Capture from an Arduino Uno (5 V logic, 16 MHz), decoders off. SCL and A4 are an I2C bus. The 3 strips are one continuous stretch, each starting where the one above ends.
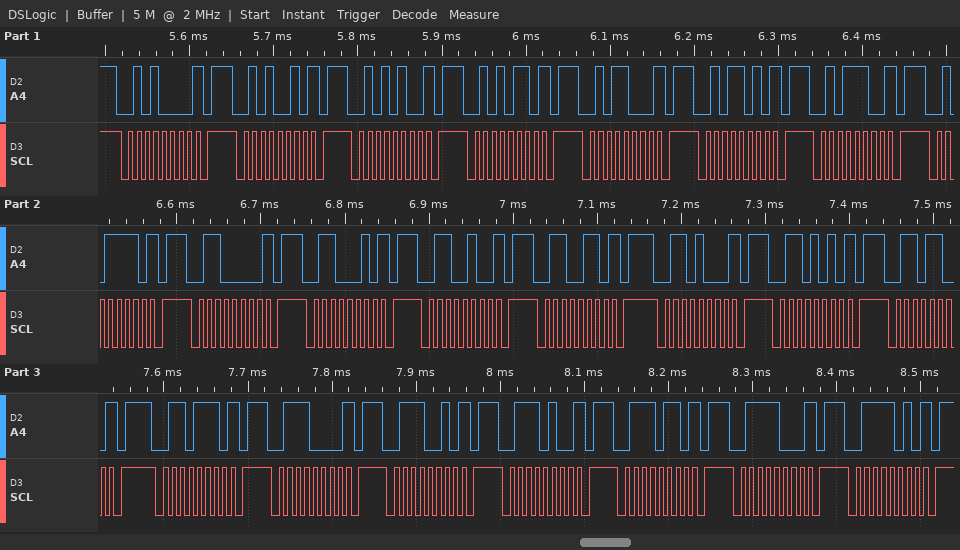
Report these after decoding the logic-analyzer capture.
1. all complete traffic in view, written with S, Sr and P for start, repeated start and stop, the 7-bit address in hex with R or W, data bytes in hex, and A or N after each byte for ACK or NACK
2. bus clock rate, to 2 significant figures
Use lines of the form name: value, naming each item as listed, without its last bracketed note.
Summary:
all complete traffic in view, written with S, Sr and P for start, repeated start and stop, the 7-bit address in hex with R or W, data bytes in hex, and A or N after each byte for ACK or NACK: S 28W N P S 29W N P S 2AW N P S 2BW N P S 2CW N P S 2DW N P S 2EW N P S 2FW N P S 30W N P S 31W N P S 32W N P S 33W N P S 34W N P S 35W N P S 36W N P S 37W N P S 38W N P S 39W N P S 3AW N P S 3BW N P S 3CW N P S 3DW N P
bus clock rate, to 2 significant figures: 100 kHz
